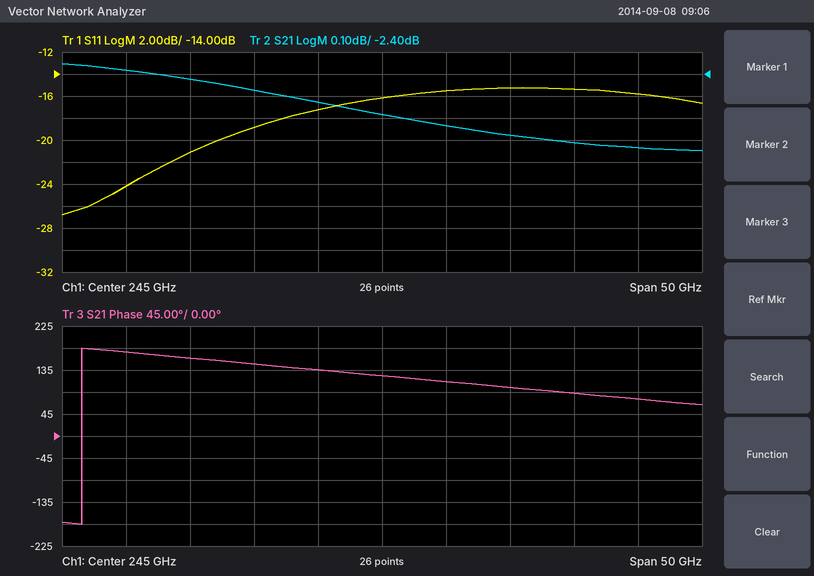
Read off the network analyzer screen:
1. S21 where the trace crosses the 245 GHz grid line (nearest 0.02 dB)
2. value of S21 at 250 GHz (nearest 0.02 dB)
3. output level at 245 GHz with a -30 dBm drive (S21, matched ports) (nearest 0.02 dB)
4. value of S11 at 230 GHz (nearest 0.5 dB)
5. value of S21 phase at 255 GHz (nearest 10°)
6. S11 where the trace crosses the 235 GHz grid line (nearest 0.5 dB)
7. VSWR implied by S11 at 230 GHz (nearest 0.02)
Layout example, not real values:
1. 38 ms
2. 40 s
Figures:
1. -2.58 dB
2. -2.64 dB
3. -32.58 dBm
4. -21.0 dB
5. 100°
6. -19.0 dB
7. 1.20
